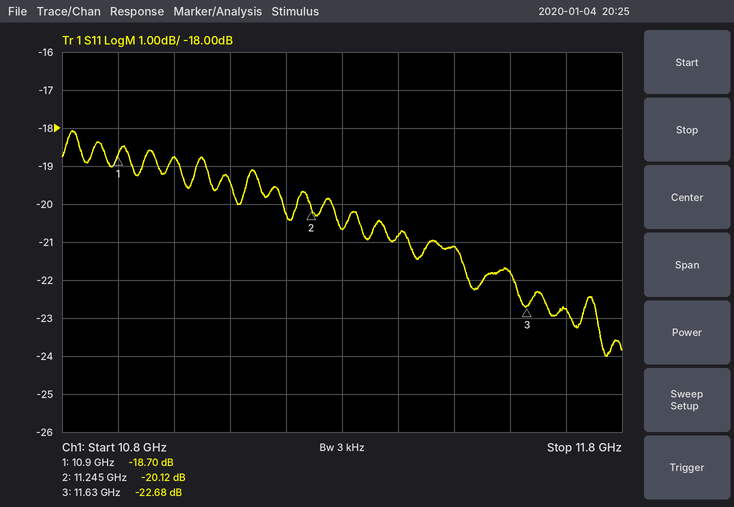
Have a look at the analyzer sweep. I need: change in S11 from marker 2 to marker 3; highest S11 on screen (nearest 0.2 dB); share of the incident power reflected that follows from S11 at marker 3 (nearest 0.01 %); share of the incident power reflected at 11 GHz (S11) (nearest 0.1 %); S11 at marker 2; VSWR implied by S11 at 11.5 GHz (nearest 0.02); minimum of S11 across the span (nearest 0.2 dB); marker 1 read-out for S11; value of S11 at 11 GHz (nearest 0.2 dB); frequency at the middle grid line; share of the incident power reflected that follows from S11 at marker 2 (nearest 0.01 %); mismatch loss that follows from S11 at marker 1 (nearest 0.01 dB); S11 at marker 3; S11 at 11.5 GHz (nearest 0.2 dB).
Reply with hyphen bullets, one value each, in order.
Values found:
- -2.56 dB
- -18.0 dB
- 0.54 %
- 1.3 %
- -20.12 dB
- 1.20
- -24.0 dB
- -18.70 dB
- -18.8 dB
- 11.3 GHz
- 0.97 %
- 0.06 dB
- -22.68 dB
- -21.2 dB
